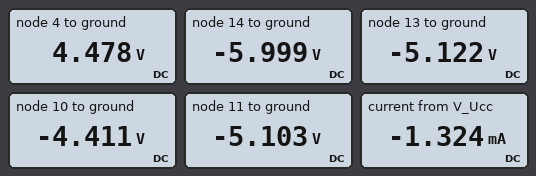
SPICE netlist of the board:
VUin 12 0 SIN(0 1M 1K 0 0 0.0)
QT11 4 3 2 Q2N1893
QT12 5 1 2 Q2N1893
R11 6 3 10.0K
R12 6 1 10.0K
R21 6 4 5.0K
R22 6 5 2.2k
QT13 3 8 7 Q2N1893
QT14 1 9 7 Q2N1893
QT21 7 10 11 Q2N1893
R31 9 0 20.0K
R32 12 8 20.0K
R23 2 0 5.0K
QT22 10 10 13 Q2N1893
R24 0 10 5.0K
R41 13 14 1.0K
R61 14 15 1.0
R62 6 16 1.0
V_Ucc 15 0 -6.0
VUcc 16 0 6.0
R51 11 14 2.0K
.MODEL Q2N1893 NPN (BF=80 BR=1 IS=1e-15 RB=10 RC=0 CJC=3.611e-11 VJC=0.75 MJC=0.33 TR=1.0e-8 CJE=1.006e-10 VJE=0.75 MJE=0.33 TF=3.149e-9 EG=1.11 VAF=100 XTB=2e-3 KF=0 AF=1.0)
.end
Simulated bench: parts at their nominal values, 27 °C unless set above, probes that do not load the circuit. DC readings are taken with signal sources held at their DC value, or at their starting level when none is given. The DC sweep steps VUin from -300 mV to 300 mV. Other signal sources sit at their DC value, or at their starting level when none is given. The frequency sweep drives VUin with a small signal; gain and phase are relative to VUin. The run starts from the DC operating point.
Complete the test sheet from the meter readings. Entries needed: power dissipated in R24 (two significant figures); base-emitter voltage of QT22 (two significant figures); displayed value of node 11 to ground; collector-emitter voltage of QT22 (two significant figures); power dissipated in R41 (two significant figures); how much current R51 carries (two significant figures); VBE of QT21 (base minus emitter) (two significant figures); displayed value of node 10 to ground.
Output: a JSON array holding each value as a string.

["3.9 mW", "710 mV", "-5.103 V", "710 mV", "770 µW", "450 µA", "690 mV", "-4.411 V"]
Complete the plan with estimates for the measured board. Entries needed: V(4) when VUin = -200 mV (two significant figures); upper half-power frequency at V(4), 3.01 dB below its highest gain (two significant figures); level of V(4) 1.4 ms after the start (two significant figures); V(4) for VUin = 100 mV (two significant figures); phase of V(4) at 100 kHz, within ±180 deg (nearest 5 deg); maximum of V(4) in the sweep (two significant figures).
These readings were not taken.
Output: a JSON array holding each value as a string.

["3.5 V", "15 kHz", "4.7 V", "6.0 V", "-110 deg", "6.0 V"]
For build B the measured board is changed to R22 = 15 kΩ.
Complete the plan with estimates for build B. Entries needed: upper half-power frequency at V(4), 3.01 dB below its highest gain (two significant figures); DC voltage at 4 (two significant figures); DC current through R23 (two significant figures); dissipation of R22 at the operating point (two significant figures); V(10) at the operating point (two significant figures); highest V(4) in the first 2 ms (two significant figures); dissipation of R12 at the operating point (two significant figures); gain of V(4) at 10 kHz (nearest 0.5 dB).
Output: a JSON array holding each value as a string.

["61 kHz", "3.9 V", "610 µA", "530 µW", "-4.4 V", "4.0 V", "510 µW", "30.5 dB"]
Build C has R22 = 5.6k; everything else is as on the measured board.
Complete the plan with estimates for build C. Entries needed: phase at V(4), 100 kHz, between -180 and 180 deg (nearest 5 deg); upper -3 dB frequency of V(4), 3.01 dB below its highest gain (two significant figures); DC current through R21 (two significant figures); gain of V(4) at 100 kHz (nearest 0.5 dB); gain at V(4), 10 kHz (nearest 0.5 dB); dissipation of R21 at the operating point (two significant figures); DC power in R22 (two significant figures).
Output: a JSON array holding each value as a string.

["-115 deg", "12 kHz", "310 µA", "30.5 dB", "48.0 dB", "470 µW", "520 µW"]
